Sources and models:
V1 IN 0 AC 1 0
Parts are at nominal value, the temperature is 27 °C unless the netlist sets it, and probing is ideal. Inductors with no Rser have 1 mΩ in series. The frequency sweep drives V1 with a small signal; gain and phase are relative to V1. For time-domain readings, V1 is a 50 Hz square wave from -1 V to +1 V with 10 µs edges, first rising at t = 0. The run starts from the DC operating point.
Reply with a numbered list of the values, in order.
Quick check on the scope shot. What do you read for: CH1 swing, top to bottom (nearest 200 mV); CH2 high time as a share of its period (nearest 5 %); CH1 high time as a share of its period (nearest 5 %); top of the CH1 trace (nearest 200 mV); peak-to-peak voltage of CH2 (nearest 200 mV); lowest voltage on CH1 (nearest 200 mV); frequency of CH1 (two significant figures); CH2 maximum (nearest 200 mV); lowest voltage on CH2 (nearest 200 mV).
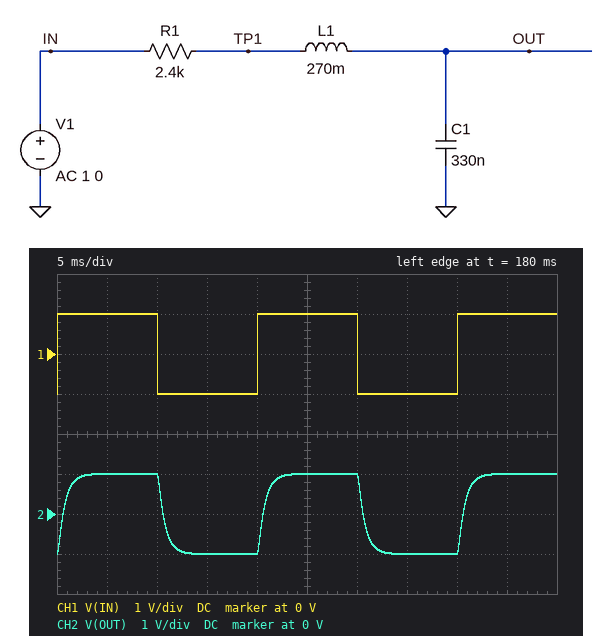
1. 2.0 V
2. 50 %
3. 50 %
4. 1.0 V
5. 2.0 V
6. -1.0 V
7. 50 Hz
8. 1.0 V
9. -1.0 V
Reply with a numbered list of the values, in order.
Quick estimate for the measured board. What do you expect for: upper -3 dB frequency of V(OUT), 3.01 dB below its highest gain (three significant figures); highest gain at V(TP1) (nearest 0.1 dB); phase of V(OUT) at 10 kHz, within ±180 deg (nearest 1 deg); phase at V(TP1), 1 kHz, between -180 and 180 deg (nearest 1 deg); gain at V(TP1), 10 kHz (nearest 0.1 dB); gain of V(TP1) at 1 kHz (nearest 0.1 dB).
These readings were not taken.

1. 233 Hz
2. 0 dB
3. -172 deg
4. 63 deg
5. -0.1 dB
6. -6.9 dB
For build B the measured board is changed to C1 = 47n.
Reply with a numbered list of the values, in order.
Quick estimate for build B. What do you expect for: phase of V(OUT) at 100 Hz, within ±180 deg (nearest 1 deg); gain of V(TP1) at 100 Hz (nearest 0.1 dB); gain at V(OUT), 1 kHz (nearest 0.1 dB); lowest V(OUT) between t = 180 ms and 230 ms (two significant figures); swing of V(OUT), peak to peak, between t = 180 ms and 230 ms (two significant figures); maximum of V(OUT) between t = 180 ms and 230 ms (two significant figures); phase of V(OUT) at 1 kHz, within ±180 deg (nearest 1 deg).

1. -4 deg
2. 0 dB
3. 1.2 dB
4. -1.3 V
5. 2.7 V
6. 1.3 V
7. -55 deg
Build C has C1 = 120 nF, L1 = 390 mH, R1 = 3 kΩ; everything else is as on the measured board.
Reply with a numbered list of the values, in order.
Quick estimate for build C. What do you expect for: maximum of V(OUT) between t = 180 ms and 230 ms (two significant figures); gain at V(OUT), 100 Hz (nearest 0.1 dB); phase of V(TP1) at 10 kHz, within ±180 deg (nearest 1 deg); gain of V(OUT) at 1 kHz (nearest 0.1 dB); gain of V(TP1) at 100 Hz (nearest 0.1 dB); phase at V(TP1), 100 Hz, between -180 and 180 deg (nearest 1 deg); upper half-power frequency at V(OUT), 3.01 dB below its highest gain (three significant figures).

1. 1.0 V
2. -0.1 dB
3. 7 deg
4. -7.7 dB
5. -0.2 dB
6. -13 deg
7. 610 Hz
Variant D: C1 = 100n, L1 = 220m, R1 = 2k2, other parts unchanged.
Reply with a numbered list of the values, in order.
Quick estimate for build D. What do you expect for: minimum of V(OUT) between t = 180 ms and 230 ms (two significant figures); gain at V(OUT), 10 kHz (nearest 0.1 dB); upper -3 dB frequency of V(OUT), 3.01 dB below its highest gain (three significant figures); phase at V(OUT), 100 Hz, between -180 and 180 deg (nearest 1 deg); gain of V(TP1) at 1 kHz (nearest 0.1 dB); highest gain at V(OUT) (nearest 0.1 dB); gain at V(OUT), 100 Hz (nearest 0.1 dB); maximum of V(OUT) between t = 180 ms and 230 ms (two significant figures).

1. -1.1 V
2. -38.8 dB
3. 1.02 kHz
4. -8 deg
5. -20.5 dB
6. 0 dB
7. 0 dB
8. 1.1 V
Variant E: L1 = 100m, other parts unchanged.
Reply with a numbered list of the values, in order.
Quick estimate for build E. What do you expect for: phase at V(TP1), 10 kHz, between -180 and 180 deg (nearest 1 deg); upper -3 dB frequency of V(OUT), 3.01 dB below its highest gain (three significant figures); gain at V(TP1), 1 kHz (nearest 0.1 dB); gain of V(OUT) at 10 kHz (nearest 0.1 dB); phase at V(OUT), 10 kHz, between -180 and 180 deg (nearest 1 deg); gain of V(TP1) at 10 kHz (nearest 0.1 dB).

1. 21 deg
2. 212 Hz
3. -24.3 dB
4. -42.8 dB
5. -159 deg
6. -0.6 dB
